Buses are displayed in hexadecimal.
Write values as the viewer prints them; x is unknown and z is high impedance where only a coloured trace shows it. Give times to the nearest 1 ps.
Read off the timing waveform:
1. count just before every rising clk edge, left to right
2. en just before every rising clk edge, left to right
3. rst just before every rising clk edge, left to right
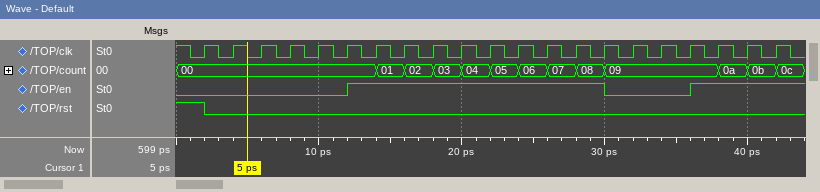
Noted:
00, 00, 00, 00, 00, 00, 00, 01, 02, 03, 04, 05, 06, 07, 08, 09, 09, 09, 09, 0a, 0b
0 0 0 0 0 0 1 1 1 1 1 1 1 1 1 0 0 0 1 1 1
1 0 0 0 0 0 0 0 0 0 0 0 0 0 0 0 0 0 0 0 0
